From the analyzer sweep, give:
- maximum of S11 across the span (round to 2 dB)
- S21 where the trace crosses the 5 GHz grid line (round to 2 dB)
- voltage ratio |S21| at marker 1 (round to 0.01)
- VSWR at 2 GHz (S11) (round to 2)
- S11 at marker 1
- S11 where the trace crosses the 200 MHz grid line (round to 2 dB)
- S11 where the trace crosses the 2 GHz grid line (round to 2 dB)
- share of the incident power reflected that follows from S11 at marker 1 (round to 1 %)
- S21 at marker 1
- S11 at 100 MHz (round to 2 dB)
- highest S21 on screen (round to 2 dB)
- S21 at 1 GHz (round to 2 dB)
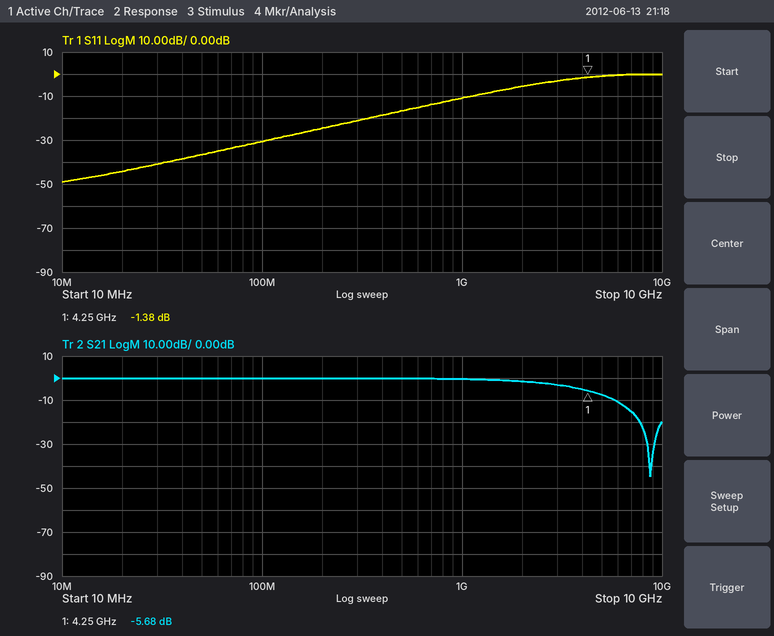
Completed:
0 dB
-8 dB
0.52
4
-1.38 dB
-24 dB
-6 dB
73 %
-5.68 dB
-30 dB
0 dB
0 dB
